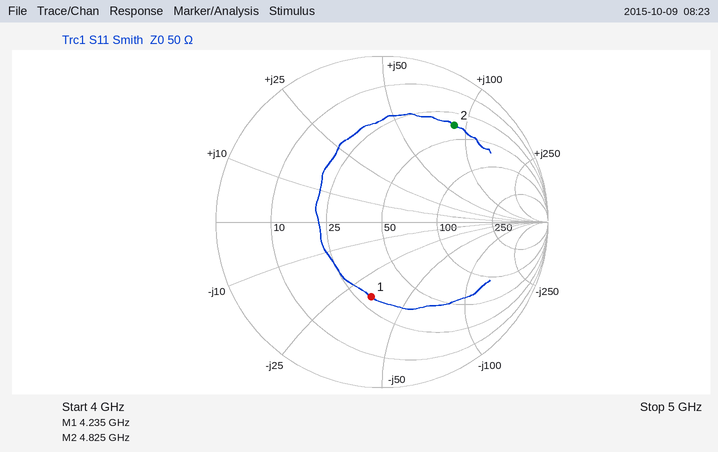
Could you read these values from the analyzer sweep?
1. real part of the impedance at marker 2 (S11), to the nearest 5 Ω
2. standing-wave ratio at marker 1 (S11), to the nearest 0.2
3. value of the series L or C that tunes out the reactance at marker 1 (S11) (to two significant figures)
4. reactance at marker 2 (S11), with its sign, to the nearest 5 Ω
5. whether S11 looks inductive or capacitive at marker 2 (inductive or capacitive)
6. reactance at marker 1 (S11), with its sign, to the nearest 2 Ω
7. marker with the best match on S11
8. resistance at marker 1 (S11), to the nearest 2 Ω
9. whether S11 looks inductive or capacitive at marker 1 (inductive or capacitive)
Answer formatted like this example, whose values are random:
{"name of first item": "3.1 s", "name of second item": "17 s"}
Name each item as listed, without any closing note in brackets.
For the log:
{"real part of the impedance at marker 2 (S11), to the nearest 5 Ω": "35 Ω", "standing-wave ratio at marker 1 (S11), to the nearest 0.2": "2.6", "value of the series L or C that tunes out the reactance at marker 1 (S11)": "1.3 nH", "reactance at marker 2 (S11), with its sign, to the nearest 5 Ω": "+90 Ω", "whether S11 looks inductive or capacitive at marker 2": "inductive", "reactance at marker 1 (S11), with its sign, to the nearest 2 Ω": "-34 Ω", "marker with the best match on S11": "marker 1", "resistance at marker 1 (S11), to the nearest 2 Ω": "30 Ω", "whether S11 looks inductive or capacitive at marker 1": "capacitive"}
